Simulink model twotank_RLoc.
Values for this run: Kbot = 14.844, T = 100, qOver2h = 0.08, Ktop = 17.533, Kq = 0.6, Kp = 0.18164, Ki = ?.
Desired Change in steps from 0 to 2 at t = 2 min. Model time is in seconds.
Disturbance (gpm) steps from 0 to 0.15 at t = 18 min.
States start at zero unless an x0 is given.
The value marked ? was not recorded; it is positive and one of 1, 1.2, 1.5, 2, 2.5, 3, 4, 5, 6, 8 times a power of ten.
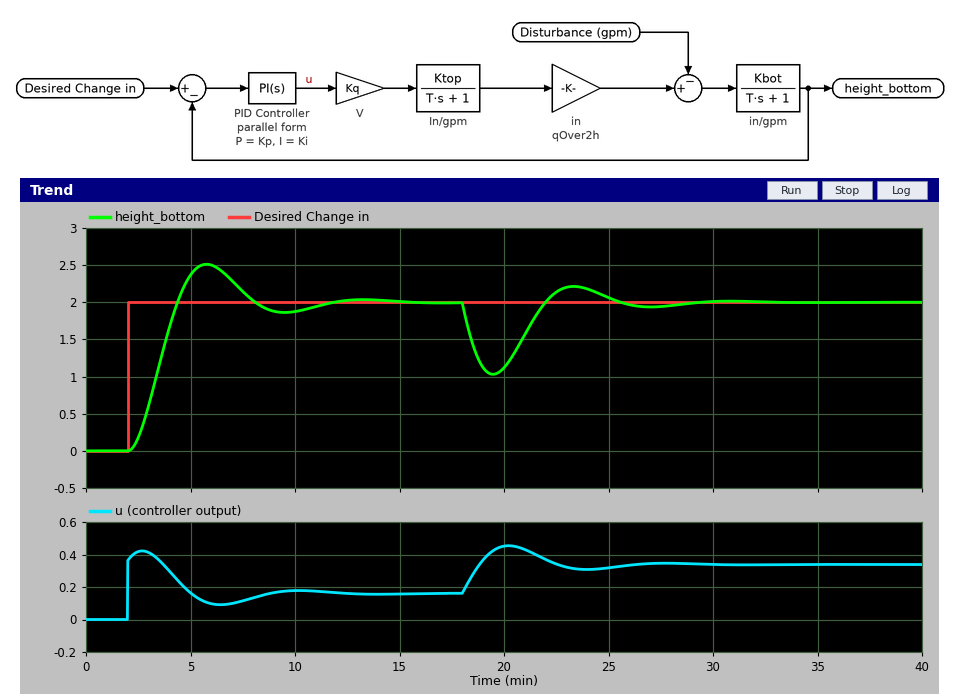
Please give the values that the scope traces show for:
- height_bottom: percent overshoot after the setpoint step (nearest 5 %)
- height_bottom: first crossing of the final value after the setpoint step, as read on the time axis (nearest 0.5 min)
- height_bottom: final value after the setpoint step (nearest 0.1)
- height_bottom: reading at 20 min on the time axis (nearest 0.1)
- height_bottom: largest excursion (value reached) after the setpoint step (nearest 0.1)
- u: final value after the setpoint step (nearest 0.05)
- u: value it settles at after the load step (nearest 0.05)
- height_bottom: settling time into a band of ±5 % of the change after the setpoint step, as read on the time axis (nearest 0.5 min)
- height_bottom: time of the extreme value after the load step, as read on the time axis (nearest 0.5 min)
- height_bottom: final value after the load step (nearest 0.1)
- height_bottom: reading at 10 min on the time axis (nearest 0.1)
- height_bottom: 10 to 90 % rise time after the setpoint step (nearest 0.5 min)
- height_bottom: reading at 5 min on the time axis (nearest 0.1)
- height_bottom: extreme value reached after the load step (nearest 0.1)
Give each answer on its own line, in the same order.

25 %
4.5 min
2.0
1.1
2.5
0.15
0.35
10.5 min
19.5 min
2.0
1.9
1.5 min
2.4
1.0
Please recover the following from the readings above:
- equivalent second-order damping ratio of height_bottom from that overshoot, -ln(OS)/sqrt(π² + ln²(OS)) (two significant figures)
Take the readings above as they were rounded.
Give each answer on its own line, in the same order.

0.40
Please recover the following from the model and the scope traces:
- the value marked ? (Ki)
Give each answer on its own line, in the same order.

0.0015
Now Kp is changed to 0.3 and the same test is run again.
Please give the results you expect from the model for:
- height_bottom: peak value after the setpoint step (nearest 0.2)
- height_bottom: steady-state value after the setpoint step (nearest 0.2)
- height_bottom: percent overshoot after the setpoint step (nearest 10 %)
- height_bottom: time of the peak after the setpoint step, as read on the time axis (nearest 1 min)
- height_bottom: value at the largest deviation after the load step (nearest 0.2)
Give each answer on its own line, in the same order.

2.4
2.0
20 %
5 min
1.2
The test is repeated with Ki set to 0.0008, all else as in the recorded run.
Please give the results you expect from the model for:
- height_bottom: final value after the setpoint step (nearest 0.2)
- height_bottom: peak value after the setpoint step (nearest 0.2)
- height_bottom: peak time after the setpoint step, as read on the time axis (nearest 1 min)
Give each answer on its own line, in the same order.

2.0
2.2
6 min
